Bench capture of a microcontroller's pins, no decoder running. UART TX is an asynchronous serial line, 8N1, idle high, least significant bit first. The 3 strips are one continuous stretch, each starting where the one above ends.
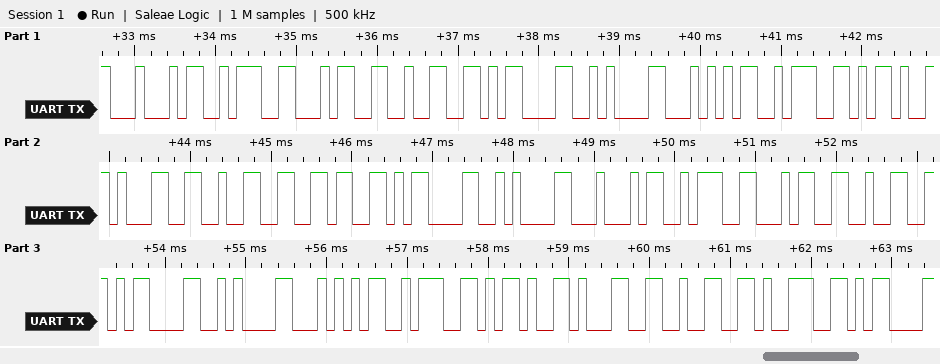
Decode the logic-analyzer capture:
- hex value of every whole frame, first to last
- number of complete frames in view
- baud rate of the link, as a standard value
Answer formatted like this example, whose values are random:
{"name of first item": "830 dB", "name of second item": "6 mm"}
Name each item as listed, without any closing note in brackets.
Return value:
{"hex value of every whole frame, first to last": "44 3A 34 32 0D 0A 54 3A 2D 31 32 36 0D 0A 44 3A 34 32 0D 0A 54 3A 2D 31 32 39 0D", "number of complete frames in view": "27", "baud rate of the link, as a standard value": "9600 baud"}
